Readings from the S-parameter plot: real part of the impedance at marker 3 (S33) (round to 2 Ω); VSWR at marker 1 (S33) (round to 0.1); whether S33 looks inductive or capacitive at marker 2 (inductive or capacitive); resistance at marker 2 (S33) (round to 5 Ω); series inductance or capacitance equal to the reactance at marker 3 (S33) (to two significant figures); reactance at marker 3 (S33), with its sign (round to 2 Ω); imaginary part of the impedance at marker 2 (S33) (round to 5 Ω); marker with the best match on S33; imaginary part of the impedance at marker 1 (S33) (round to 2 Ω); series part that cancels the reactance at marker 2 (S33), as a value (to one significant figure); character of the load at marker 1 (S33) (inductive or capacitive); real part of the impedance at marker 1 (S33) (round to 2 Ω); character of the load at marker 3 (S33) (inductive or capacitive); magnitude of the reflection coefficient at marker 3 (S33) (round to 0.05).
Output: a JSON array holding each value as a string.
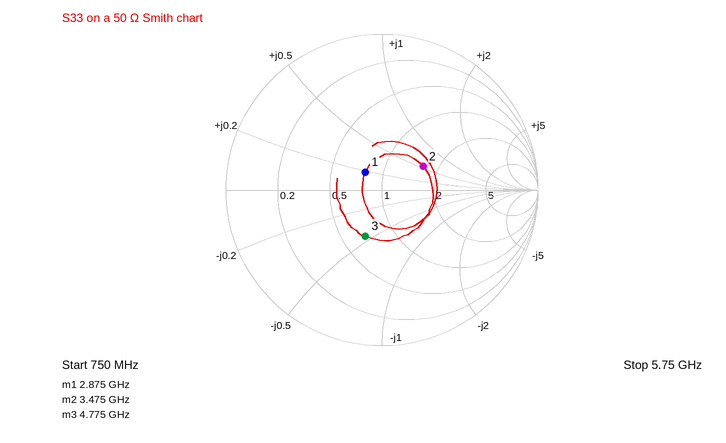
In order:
["34 Ω", "1.4", "inductive", "80 Ω", "1.5 pF", "-22 Ω", "+25 Ω", "marker 1", "+10 Ω", "2 pF", "inductive", "40 Ω", "capacitive", "0.30"]
